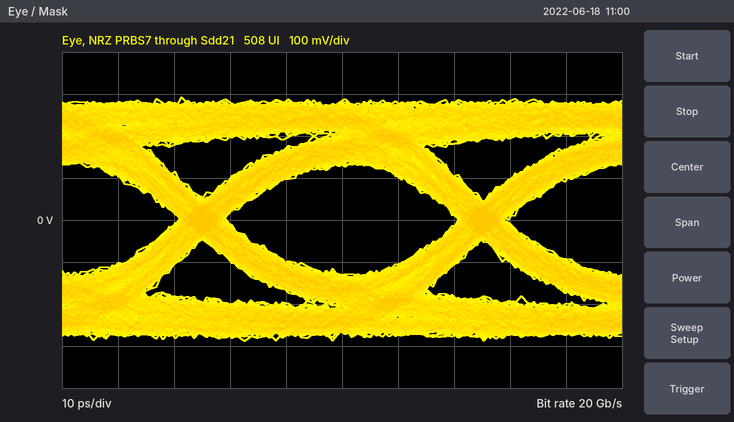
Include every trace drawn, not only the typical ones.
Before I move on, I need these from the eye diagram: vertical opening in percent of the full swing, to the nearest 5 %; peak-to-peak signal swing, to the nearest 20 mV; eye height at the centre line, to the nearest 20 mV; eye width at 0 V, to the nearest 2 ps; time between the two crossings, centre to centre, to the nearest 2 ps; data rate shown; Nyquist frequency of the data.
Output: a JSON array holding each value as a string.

["45 %", "580 mV", "260 mV", "42 ps", "50 ps", "20 Gb/s", "10 GHz"]
